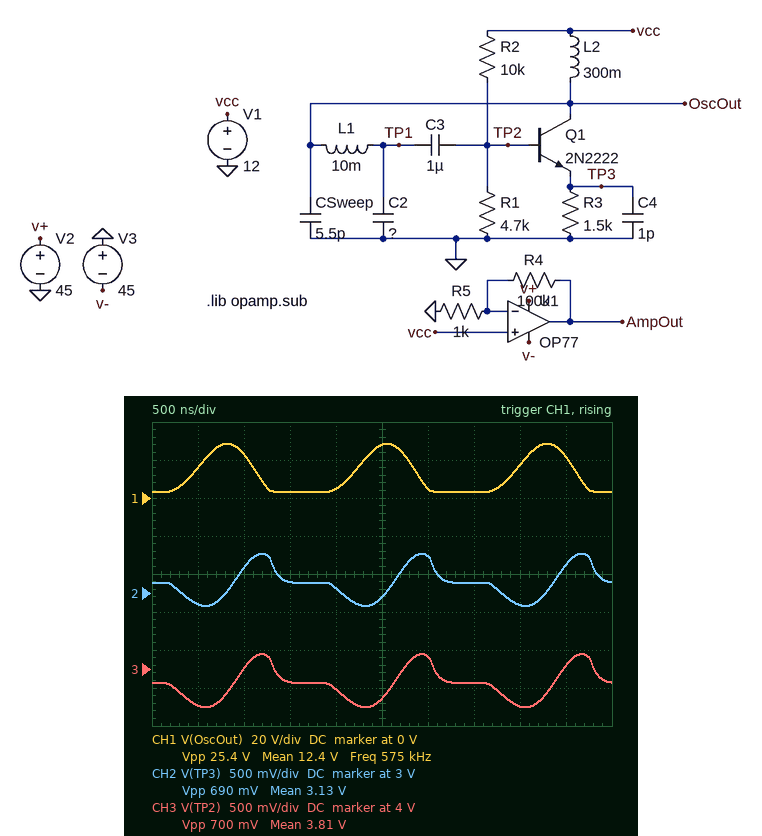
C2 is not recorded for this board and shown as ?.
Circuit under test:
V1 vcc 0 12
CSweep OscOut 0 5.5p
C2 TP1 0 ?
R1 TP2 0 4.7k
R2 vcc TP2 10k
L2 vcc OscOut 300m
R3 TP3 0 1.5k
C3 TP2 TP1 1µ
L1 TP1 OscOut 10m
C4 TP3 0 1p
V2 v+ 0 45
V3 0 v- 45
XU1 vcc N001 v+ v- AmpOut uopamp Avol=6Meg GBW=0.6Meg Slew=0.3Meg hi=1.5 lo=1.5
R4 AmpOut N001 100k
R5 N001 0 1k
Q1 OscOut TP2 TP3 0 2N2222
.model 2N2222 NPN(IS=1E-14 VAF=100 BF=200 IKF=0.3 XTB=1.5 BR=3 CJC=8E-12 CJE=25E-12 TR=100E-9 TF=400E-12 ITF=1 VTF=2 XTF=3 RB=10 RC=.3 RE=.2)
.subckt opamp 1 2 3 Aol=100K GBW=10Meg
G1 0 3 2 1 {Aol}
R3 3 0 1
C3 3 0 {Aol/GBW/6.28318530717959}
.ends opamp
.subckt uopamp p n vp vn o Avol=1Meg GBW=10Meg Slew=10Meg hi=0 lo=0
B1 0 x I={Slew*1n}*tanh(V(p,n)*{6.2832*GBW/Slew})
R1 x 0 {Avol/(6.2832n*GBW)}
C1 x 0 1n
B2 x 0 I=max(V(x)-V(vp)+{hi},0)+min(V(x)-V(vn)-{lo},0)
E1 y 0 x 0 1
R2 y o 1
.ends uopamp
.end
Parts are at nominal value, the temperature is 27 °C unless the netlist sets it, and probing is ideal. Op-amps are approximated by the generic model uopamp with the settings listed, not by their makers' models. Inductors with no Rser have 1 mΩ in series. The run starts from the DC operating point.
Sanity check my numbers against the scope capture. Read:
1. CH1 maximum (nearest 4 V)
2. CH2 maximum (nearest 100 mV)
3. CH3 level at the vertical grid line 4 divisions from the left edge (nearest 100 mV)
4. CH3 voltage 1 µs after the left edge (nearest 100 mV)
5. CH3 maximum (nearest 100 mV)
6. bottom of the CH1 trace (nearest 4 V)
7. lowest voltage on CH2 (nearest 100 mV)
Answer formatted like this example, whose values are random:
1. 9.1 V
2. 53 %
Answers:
1. 28 V
2. 3.5 V
3. 3.7 V
4. 4.0 V
5. 4.2 V
6. 4 V
7. 2.8 V
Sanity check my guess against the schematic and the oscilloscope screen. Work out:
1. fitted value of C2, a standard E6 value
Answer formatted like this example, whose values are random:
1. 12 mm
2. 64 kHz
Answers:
1. 68 pF
